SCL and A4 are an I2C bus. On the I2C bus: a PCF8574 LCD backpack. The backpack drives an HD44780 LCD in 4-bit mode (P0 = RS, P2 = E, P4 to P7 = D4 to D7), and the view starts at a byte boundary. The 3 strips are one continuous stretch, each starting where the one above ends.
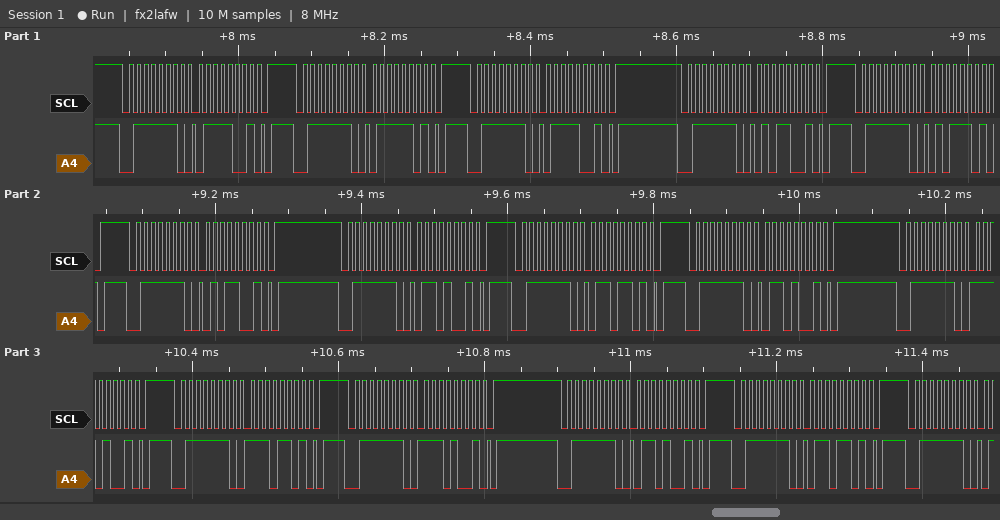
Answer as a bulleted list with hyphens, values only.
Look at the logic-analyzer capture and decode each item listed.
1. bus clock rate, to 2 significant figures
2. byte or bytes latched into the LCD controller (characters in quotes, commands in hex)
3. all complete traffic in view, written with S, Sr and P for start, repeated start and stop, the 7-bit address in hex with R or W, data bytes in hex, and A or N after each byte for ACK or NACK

- 100 kHz
- 'u' 'n'
- S 3FW A 79 A P S 3FW A 7D A P S 3FW A 79 A P S 3FW A 59 A P S 3FW A 5D A P S 3FW A 59 A P S 3FW A 69 A P S 3FW A 6D A P S 3FW A 69 A P S 3FW A E9 A P S 3FW A ED A P S 3FW A E9 A P S 3FW A 69 A P S 3FW A 6D A P S 3FW A
